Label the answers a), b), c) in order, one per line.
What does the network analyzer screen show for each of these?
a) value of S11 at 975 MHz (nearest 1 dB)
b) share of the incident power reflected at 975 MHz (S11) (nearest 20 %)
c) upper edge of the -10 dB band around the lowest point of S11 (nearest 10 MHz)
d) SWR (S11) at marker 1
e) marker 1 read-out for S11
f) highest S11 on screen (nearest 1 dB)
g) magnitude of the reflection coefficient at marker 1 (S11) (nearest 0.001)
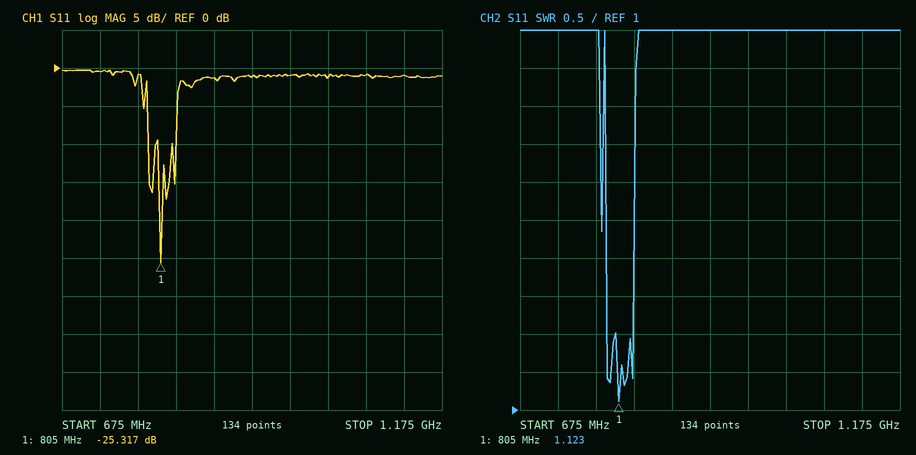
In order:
a) -1 dB
b) 80 %
c) 820 MHz
d) 1.123
e) -25.317 dB
f) 0 dB
g) 0.054
